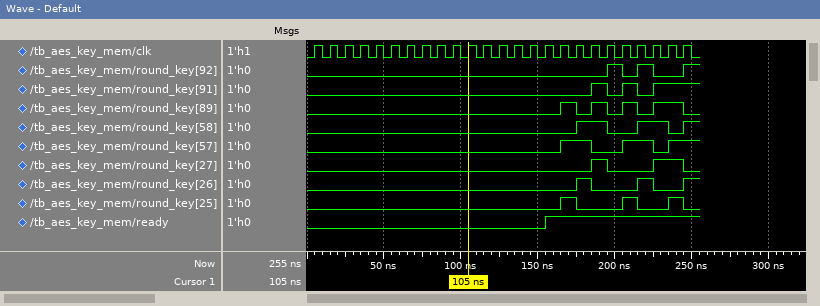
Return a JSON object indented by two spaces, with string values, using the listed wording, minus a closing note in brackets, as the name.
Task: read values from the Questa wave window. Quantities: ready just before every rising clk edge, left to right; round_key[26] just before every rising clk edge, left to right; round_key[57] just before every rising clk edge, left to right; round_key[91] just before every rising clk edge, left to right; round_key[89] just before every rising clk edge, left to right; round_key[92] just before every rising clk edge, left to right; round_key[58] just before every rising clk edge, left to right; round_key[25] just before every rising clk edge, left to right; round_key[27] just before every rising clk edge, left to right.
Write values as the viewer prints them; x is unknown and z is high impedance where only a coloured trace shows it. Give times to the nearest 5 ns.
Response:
{
  "ready just before every rising clk edge, left to right": "0 0 0 0 0 0 0 0 0 0 0 0 0 0 0 0 1 1 1 1 1 1 1 1 1",
  "round_key[26] just before every rising clk edge, left to right": "0 0 0 0 0 0 0 0 0 0 0 0 0 0 0 0 0 0 1 0 0 0 1 0 0",
  "round_key[57] just before every rising clk edge, left to right": "0 0 0 0 0 0 0 0 0 0 0 0 0 0 0 0 0 1 1 0 0 1 1 0 1",
  "round_key[91] just before every rising clk edge, left to right": "0 0 0 0 0 0 0 0 0 0 0 0 0 0 0 0 0 0 0 1 0 1 0 1 1",
  "round_key[89] just before every rising clk edge, left to right": "0 0 0 0 0 0 0 0 0 0 0 0 0 0 0 0 0 1 0 1 0 1 0 1 1",
  "round_key[92] just before every rising clk edge, left to right": "0 0 0 0 0 0 0 0 0 0 0 0 0 0 0 0 0 0 0 0 1 0 1 0 0",
  "round_key[58] just before every rising clk edge, left to right": "0 0 0 0 0 0 0 0 0 0 0 0 0 0 0 0 0 0 1 1 0 0 1 1 0",
  "round_key[25] just before every rising clk edge, left to right": "0 0 0 0 0 0 0 0 0 0 0 0 0 0 0 0 0 1 0 0 0 1 0 0 1",
  "round_key[27] just before every rising clk edge, left to right": "0 0 0 0 0 0 0 0 0 0 0 0 0 0 0 0 0 0 0 1 0 0 0 1 1"
}
